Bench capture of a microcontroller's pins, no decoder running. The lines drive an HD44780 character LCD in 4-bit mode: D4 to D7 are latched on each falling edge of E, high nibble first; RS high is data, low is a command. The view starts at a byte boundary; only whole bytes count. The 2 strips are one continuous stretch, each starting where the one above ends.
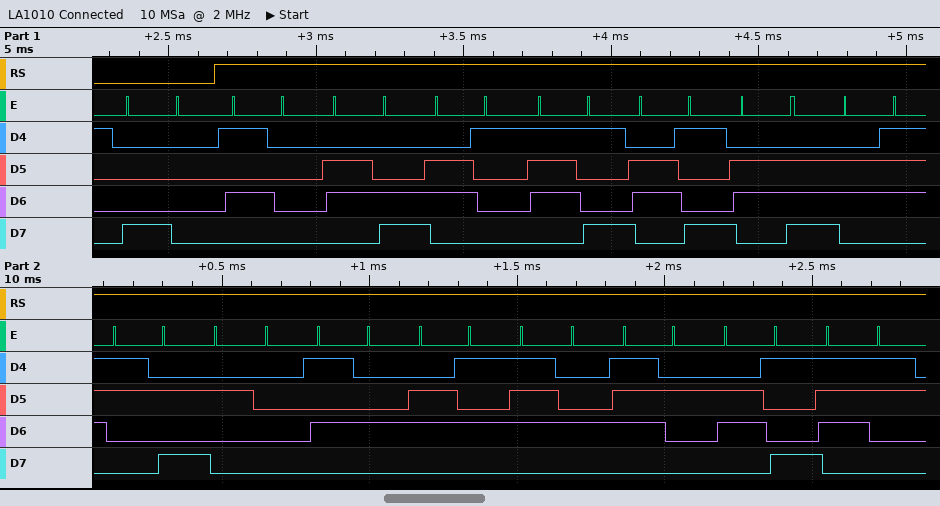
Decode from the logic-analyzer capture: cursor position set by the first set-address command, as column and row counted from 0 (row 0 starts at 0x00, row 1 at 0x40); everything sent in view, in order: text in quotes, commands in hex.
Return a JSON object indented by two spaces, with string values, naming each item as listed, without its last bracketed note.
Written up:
{
  "cursor position set by the first set-address command, as column and row counted from 0": "column 0, row 0",
  "everything sent in view, in order: text in quotes, commands in hex": "0x80 \"Playing: Tetris\""
}
